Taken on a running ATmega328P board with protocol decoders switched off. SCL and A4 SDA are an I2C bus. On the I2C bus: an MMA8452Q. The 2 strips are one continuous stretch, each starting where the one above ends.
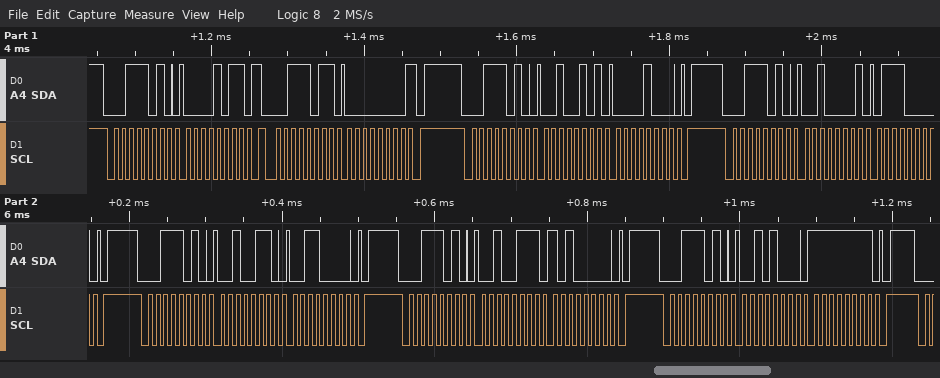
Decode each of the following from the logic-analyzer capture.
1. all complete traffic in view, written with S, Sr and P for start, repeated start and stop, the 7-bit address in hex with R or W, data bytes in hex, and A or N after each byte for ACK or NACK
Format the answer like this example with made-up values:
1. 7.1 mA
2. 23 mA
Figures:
1. S 1DW A 0B A Sr 1DR A 00 N P S 1DW A 25 A 08 A P S 1DW A 21 A 70 A P S 1DW A 26 A 30 A P S 1DW A 27 A A0 A P S 1DW A 28 A FF A P
